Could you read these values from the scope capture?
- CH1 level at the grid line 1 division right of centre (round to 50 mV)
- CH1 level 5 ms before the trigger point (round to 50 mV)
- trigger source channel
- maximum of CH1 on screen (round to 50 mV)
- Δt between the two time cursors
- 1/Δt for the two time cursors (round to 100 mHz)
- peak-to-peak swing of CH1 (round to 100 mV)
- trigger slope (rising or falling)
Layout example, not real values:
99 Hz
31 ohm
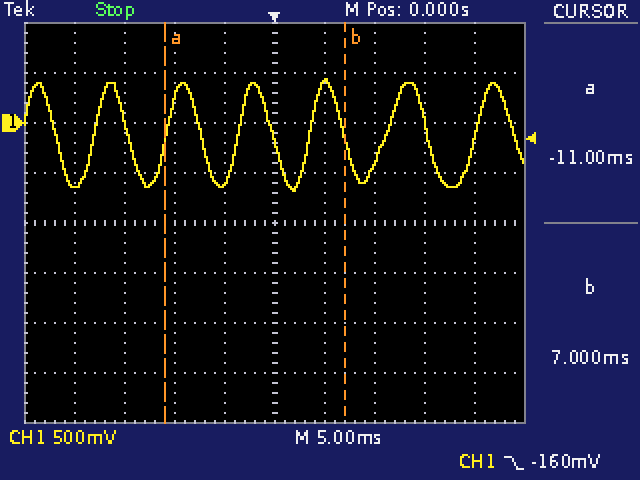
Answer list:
400 mV
-600 mV
CH1
450 mV
18.0 ms
55.6 Hz
1.10 V
falling
